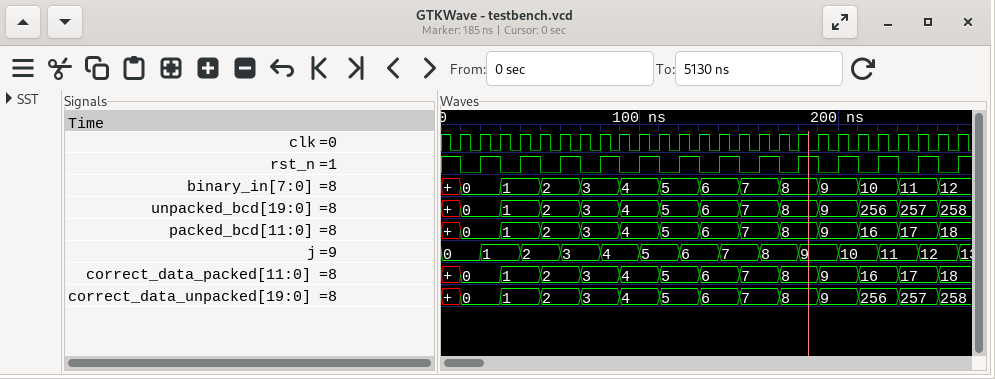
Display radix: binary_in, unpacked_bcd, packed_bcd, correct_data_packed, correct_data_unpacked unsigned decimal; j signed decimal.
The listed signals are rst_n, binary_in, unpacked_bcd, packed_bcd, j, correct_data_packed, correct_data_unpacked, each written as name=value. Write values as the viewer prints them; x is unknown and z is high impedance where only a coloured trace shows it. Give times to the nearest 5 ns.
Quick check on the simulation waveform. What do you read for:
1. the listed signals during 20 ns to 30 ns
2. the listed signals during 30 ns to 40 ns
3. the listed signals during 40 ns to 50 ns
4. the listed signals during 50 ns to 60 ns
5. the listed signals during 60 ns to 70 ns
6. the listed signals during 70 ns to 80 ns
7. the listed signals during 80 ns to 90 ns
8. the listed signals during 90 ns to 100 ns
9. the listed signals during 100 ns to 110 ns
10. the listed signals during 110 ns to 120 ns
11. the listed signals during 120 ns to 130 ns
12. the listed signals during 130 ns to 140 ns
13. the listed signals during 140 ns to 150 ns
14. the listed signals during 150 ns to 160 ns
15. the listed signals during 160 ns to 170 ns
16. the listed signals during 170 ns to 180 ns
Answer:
rst_n=1, binary_in=0, unpacked_bcd=0, packed_bcd=0, j=1, correct_data_packed=0, correct_data_unpacked=0
rst_n=0, binary_in=1, unpacked_bcd=1, packed_bcd=1, j=1, correct_data_packed=1, correct_data_unpacked=1
rst_n=1, binary_in=1, unpacked_bcd=1, packed_bcd=1, j=2, correct_data_packed=1, correct_data_unpacked=1
rst_n=0, binary_in=2, unpacked_bcd=2, packed_bcd=2, j=2, correct_data_packed=2, correct_data_unpacked=2
rst_n=1, binary_in=2, unpacked_bcd=2, packed_bcd=2, j=3, correct_data_packed=2, correct_data_unpacked=2
rst_n=0, binary_in=3, unpacked_bcd=3, packed_bcd=3, j=3, correct_data_packed=3, correct_data_unpacked=3
rst_n=1, binary_in=3, unpacked_bcd=3, packed_bcd=3, j=4, correct_data_packed=3, correct_data_unpacked=3
rst_n=0, binary_in=4, unpacked_bcd=4, packed_bcd=4, j=4, correct_data_packed=4, correct_data_unpacked=4
rst_n=1, binary_in=4, unpacked_bcd=4, packed_bcd=4, j=5, correct_data_packed=4, correct_data_unpacked=4
rst_n=0, binary_in=5, unpacked_bcd=5, packed_bcd=5, j=5, correct_data_packed=5, correct_data_unpacked=5
rst_n=1, binary_in=5, unpacked_bcd=5, packed_bcd=5, j=6, correct_data_packed=5, correct_data_unpacked=5
rst_n=0, binary_in=6, unpacked_bcd=6, packed_bcd=6, j=6, correct_data_packed=6, correct_data_unpacked=6
rst_n=1, binary_in=6, unpacked_bcd=6, packed_bcd=6, j=7, correct_data_packed=6, correct_data_unpacked=6
rst_n=0, binary_in=7, unpacked_bcd=7, packed_bcd=7, j=7, correct_data_packed=7, correct_data_unpacked=7
rst_n=1, binary_in=7, unpacked_bcd=7, packed_bcd=7, j=8, correct_data_packed=7, correct_data_unpacked=7
rst_n=0, binary_in=8, unpacked_bcd=8, packed_bcd=8, j=8, correct_data_packed=8, correct_data_unpacked=8
